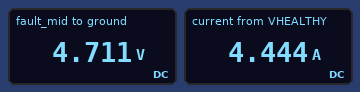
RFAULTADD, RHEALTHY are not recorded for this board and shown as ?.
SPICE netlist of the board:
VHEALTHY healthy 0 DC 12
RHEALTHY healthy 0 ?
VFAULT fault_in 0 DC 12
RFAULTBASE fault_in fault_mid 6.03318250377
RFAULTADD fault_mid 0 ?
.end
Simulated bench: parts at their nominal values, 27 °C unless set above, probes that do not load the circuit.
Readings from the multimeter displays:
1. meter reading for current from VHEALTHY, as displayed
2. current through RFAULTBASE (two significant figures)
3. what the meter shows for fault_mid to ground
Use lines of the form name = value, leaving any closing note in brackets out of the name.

meter reading for current from VHEALTHY, as displayed = 4.444 A
current through RFAULTBASE = 1.2 A
what the meter shows for fault_mid to ground = 4.711 V
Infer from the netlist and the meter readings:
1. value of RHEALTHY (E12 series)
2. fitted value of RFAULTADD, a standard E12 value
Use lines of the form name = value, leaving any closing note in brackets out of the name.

value of RHEALTHY = 2.7 Ω
fitted value of RFAULTADD, a standard E12 value = 3.9 Ω
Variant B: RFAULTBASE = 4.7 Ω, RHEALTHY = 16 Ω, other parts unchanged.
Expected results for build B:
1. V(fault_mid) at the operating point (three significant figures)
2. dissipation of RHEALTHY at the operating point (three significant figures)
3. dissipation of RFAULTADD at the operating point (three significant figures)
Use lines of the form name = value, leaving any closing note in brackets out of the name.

V(fault_mid) at the operating point = 5.44 V
dissipation of RHEALTHY at the operating point = 9.00 W
dissipation of RFAULTADD at the operating point = 7.59 W
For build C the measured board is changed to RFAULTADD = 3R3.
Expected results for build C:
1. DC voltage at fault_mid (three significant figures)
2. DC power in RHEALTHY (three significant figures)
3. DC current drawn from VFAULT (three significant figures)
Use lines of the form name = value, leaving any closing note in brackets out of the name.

DC voltage at fault_mid = 4.24 V
DC power in RHEALTHY = 53.3 W
DC current drawn from VFAULT = 1.29 A
